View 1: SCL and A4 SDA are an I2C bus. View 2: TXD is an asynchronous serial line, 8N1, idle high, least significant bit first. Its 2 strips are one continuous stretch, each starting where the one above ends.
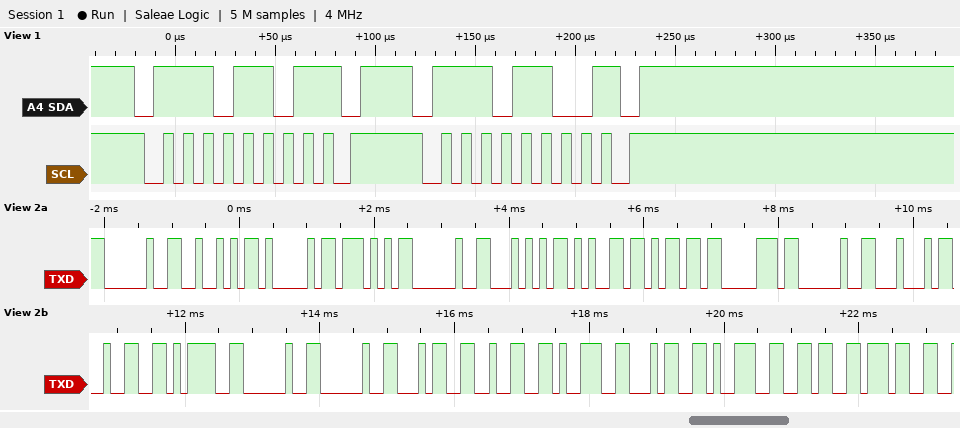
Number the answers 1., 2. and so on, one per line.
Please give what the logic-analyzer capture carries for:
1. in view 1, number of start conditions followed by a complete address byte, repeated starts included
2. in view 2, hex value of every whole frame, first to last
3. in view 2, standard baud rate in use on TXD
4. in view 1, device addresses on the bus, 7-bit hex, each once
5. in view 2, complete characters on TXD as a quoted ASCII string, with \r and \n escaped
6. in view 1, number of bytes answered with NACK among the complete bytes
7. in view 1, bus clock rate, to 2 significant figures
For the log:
1. 2
2. 0x20 0x52 0x41 0x57 0x20 0x54 0x65 0x6D 0x70 0x20 0x44 0x32 0x3D 0x20 0x20 0x34 0x32 0x39 0x34 0x39 0x36 0x37
3. 9600 baud
4. 0x76
5. " RAW Temp D2=  4294967"
6. 2
7. 100 kHz
